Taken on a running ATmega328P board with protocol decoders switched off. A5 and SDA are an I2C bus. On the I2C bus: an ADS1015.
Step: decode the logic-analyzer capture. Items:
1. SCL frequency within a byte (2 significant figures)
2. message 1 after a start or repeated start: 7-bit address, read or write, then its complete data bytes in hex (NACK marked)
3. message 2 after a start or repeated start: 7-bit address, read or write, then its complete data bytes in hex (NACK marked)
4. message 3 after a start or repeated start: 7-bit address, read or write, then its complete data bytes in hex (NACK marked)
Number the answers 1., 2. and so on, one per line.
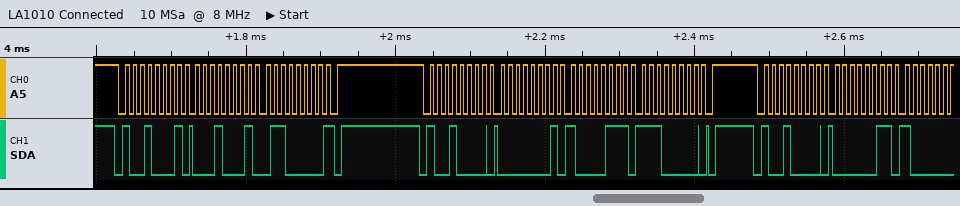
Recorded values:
1. 100 kHz
2. 0x48 read: 11 60 NACK
3. 0x48 write: 01 87 E0
4. 0x48 write: 03
